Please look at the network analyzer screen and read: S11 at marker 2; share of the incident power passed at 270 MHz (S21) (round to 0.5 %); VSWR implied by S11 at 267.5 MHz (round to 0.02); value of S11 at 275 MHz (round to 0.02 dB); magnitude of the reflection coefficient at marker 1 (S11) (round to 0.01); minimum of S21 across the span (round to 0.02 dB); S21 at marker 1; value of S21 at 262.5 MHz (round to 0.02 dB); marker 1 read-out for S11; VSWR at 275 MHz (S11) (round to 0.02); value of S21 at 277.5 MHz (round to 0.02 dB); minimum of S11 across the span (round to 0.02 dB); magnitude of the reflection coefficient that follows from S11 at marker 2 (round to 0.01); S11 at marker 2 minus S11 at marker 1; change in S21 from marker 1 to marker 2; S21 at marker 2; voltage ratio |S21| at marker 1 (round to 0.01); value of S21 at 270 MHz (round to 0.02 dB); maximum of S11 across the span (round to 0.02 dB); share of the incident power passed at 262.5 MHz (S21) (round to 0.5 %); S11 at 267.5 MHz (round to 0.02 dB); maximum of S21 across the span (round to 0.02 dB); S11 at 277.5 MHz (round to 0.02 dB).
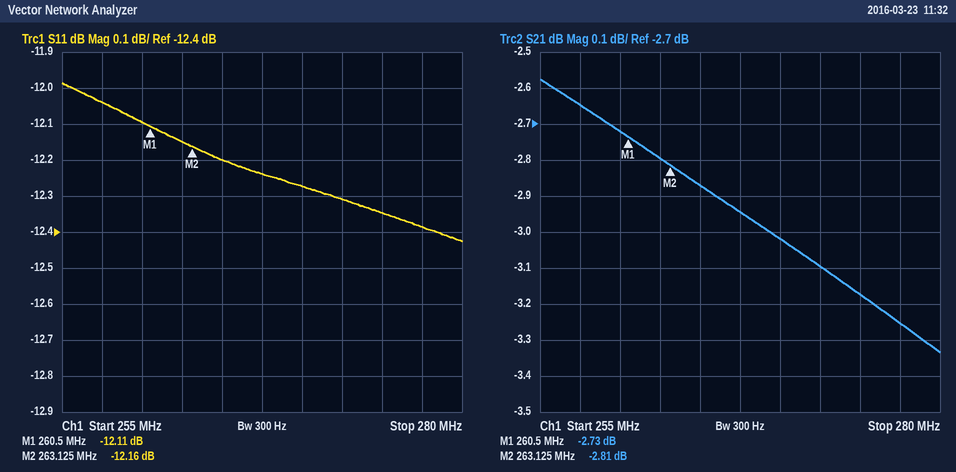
-12.16 dB
50.0 %
1.64
-12.34 dB
0.25
-3.34 dB
-2.73 dB
-2.80 dB
-12.11 dB
1.64
-3.26 dB
-12.42 dB
0.25
-0.05 dB
-0.08 dB
-2.81 dB
0.73
-3.02 dB
-11.98 dB
52.5 %
-12.24 dB
-2.58 dB
-12.38 dB
